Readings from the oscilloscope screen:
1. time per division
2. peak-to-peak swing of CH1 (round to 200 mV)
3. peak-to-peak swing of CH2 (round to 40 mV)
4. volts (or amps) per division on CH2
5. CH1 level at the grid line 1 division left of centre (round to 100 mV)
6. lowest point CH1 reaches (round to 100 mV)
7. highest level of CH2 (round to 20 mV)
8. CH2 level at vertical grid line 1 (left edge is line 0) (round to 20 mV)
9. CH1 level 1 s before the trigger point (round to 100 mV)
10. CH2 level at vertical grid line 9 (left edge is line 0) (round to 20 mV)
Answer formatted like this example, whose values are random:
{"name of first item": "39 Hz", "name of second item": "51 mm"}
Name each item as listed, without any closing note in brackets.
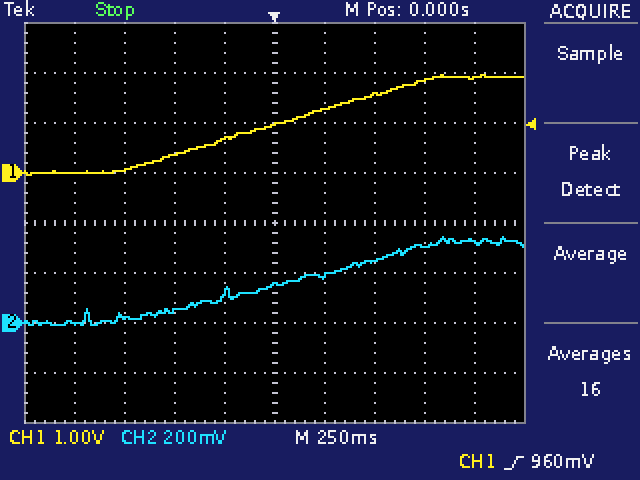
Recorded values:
{"time per division": "250 ms", "peak-to-peak swing of CH1": "2.0 V", "peak-to-peak swing of CH2": "360 mV", "volts (or amps) per division on CH2": "200 mV", "CH1 level at the grid line 1 division left of centre": "700 mV", "lowest point CH1 reaches": "0.0 V", "highest level of CH2": "340 mV", "CH2 level at vertical grid line 1 (left edge is line 0)": "0 mV", "CH1 level 1 s before the trigger point": "0.0 V", "CH2 level at vertical grid line 9 (left edge is line 0)": "320 mV"}
